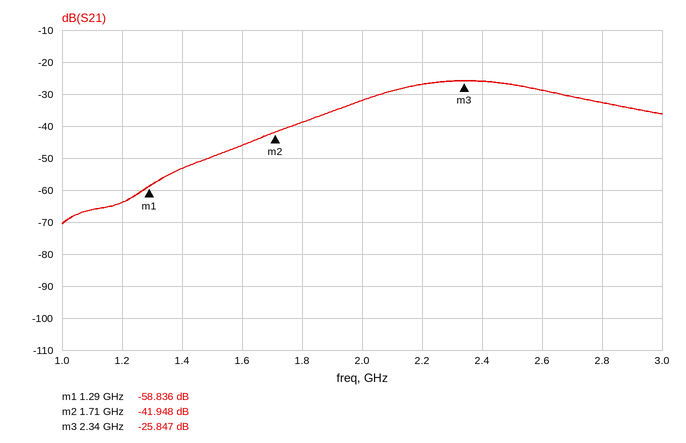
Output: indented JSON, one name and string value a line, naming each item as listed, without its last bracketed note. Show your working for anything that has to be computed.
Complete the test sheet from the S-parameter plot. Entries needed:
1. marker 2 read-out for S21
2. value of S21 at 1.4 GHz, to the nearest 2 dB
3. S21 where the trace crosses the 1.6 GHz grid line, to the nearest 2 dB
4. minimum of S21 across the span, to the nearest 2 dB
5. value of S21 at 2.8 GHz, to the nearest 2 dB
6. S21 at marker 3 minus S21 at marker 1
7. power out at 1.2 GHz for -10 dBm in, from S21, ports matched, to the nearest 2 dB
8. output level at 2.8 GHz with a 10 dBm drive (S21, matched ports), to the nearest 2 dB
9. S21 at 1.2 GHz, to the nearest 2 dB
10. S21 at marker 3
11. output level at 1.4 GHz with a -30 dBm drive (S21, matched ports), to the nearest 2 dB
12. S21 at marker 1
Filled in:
{
  "marker 2 read-out for S21": "-41.948 dB",
  "value of S21 at 1.4 GHz, to the nearest 2 dB": "-54 dB",
  "S21 where the trace crosses the 1.6 GHz grid line, to the nearest 2 dB": "-46 dB",
  "minimum of S21 across the span, to the nearest 2 dB": "-70 dB",
  "value of S21 at 2.8 GHz, to the nearest 2 dB": "-32 dB",
  "S21 at marker 3 minus S21 at marker 1": "-25.847 − (-58.836) = 32.989 dB",
  "power out at 1.2 GHz for -10 dBm in, from S21, ports matched, to the nearest 2 dB": "-10 dBm + (-64 dB) = -74 dBm",
  "output level at 2.8 GHz with a 10 dBm drive (S21, matched ports), to the nearest 2 dB": "10 dBm + (-32 dB) = -22 dBm",
  "S21 at 1.2 GHz, to the nearest 2 dB": "-64 dB",
  "S21 at marker 3": "-25.847 dB",
  "output level at 1.4 GHz with a -30 dBm drive (S21, matched ports), to the nearest 2 dB": "-30 dBm + (-54 dB) = -84 dBm",
  "S21 at marker 1": "-58.836 dB"
}
